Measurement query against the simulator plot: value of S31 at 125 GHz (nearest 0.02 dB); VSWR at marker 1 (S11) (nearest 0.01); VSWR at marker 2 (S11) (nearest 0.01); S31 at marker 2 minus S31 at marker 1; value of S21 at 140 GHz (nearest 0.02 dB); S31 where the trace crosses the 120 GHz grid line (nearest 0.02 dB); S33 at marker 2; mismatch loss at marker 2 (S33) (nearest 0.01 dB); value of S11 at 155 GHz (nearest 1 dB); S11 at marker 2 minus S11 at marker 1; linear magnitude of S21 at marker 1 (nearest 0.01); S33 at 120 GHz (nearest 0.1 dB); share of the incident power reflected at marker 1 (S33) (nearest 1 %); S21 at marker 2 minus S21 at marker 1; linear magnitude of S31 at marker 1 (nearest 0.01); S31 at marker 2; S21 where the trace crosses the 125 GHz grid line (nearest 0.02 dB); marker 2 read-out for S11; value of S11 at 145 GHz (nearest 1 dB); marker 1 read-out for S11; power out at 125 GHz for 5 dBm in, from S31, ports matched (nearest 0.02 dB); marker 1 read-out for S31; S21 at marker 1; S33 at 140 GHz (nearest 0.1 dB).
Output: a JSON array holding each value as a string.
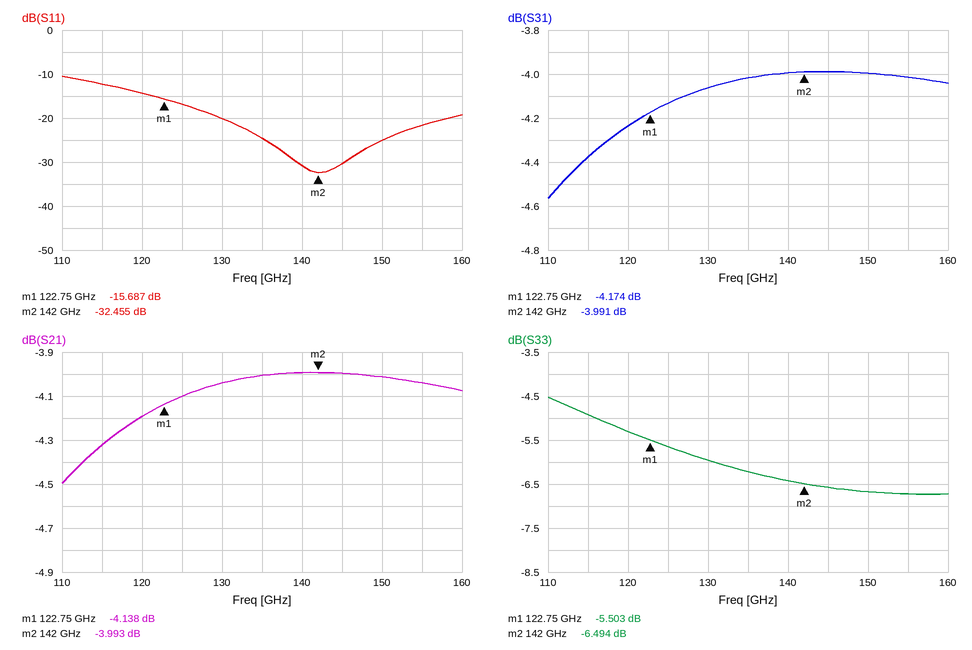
["-4.14 dB", "1.39", "1.05", "0.183 dB", "-4.00 dB", "-4.24 dB", "-6.494 dB", "1.10 dB", "-22 dB", "-16.768 dB", "0.62", "-5.3 dB", "28 %", "0.145 dB", "0.62", "-3.991 dB", "-4.10 dB", "-32.455 dB", "-30 dB", "-15.687 dB", "0.86 dBm", "-4.174 dB", "-4.138 dB", "-6.4 dB"]
